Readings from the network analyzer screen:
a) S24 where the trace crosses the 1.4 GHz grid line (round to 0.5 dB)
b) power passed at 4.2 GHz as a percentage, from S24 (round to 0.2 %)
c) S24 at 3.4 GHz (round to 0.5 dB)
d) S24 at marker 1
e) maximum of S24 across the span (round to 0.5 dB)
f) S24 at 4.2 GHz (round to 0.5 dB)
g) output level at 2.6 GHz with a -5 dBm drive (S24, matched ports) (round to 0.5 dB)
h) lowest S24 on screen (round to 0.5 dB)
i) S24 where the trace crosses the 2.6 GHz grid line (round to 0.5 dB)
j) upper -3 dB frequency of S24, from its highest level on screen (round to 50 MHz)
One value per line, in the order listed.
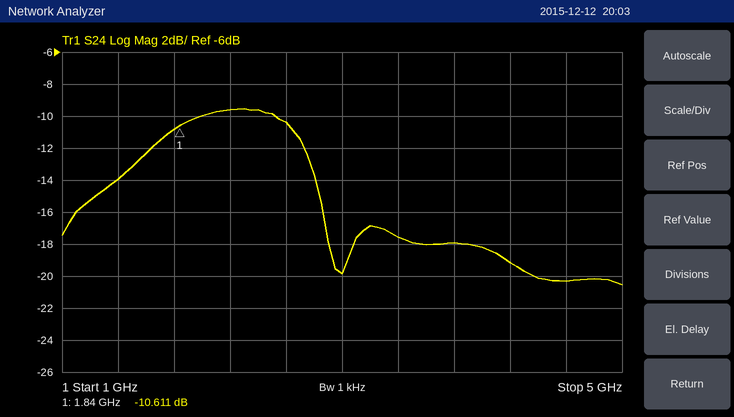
-14.0 dB
1.2 %
-17.5 dB
-10.611 dB
-9.5 dB
-19.0 dB
-15.5 dBm
-20.5 dB
-10.5 dB
2.75 GHz
